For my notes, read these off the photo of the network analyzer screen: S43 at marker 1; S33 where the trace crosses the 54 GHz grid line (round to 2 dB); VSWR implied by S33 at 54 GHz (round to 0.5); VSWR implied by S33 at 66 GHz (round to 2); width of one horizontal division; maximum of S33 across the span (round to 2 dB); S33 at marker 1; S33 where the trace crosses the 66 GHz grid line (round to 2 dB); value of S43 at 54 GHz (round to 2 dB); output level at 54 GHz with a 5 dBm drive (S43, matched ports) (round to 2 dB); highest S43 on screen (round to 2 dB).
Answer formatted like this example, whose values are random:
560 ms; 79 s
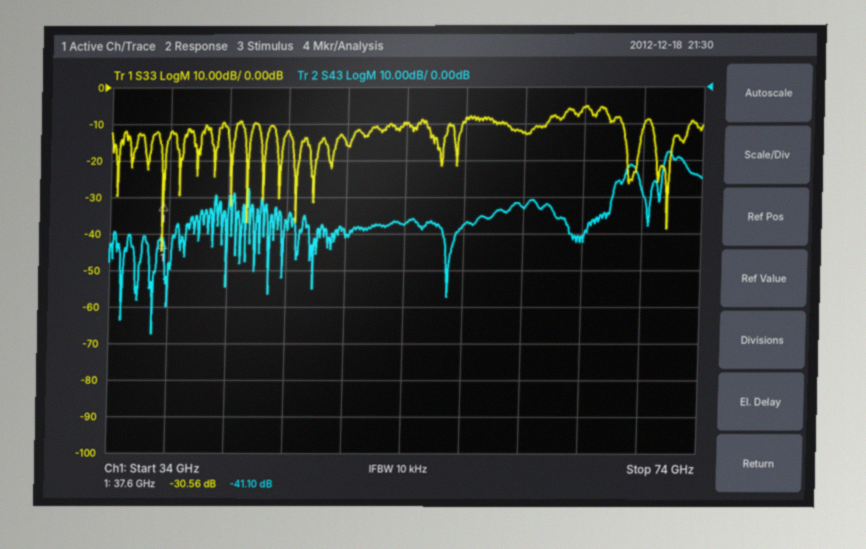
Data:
-41.10 dB; -10 dB; 2.0; 4; 4 GHz; -6 dB; -30.56 dB; -6 dB; -38 dB; -32 dBm; -18 dB
